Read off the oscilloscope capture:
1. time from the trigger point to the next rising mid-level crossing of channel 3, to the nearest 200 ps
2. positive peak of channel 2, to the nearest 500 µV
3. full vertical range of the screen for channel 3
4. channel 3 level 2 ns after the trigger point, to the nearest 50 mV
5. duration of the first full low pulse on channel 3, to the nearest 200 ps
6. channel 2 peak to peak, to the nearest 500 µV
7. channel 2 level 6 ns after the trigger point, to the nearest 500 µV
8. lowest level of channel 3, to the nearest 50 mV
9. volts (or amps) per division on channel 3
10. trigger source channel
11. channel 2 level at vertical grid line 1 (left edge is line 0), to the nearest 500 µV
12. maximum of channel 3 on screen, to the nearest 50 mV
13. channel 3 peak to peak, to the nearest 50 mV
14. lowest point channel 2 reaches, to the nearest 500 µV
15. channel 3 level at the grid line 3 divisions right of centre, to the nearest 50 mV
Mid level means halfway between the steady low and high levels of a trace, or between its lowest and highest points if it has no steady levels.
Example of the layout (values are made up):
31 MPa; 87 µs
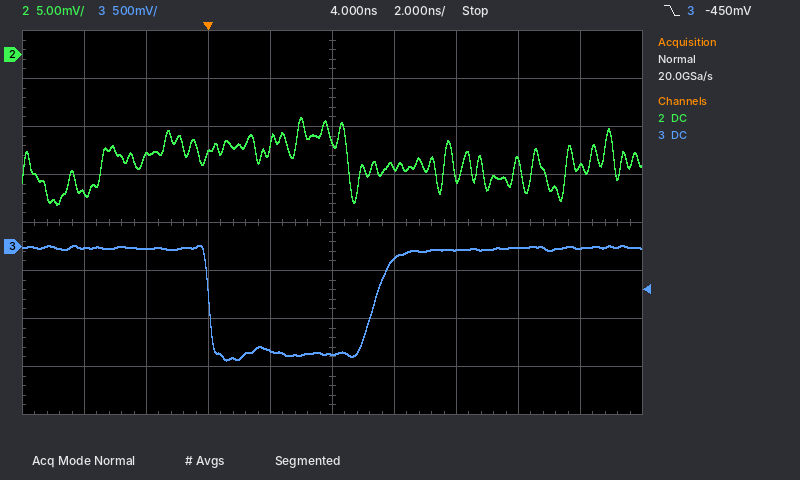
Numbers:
5.4 ns; -6.5 mV; 4 V; -1.10 V; 5.4 ns; 9.0 mV; -11.5 mV; -1.20 V; 500 mV; channel 3; -14.5 mV; 0 mV; 1.20 V; -15.5 mV; 0 mV
